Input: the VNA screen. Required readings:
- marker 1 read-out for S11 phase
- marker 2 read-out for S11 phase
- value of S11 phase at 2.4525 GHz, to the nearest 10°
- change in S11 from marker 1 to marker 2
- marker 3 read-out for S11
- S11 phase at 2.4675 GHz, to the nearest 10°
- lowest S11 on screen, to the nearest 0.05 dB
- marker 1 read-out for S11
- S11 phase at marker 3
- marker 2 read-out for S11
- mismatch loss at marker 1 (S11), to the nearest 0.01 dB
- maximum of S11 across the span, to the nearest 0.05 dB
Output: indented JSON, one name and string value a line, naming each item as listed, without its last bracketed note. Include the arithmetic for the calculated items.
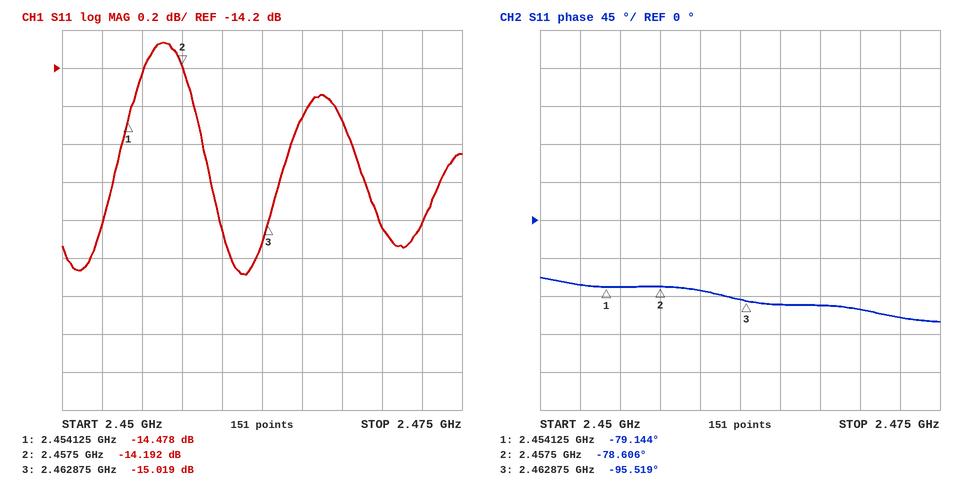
{
  "marker 1 read-out for S11 phase": "-79.144°",
  "marker 2 read-out for S11 phase": "-78.606°",
  "value of S11 phase at 2.4525 GHz, to the nearest 10°": "-80°",
  "change in S11 from marker 1 to marker 2": "-14.192 − (-14.478) = 0.286 dB",
  "marker 3 read-out for S11": "-15.019 dB",
  "S11 phase at 2.4675 GHz, to the nearest 10°": "-100°",
  "lowest S11 on screen, to the nearest 0.05 dB": "-15.30 dB",
  "marker 1 read-out for S11": "-14.478 dB",
  "S11 phase at marker 3": "-95.519°",
  "marker 2 read-out for S11": "-14.192 dB",
  "mismatch loss at marker 1 (S11), to the nearest 0.01 dB": "−10 log10(1 − 10^(-14.478/10)) ≈ 0.16 dB",
  "maximum of S11 across the span, to the nearest 0.05 dB": "-14.05 dB"
}
